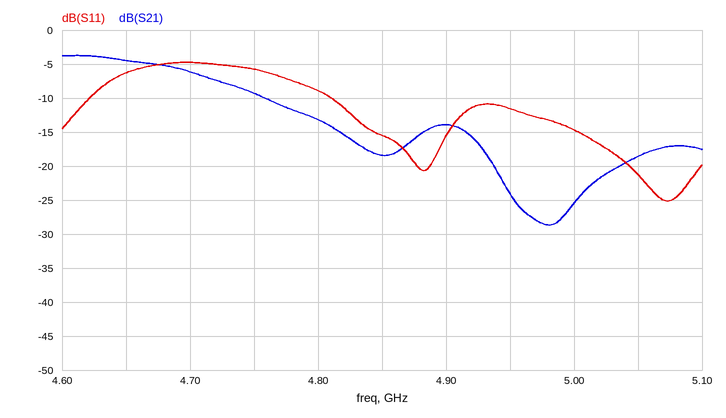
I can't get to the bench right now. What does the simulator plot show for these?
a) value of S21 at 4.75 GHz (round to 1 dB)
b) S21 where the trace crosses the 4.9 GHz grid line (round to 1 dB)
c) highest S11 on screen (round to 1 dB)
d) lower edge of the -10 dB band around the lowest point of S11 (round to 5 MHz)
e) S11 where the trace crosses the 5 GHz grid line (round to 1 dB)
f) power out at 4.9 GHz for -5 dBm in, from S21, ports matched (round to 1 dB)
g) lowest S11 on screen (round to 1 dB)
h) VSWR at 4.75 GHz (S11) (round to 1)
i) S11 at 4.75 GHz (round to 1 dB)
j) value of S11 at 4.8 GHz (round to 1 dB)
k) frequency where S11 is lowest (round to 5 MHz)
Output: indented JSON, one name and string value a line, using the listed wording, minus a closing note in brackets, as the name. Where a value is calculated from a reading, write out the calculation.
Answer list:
{
  "value of S21 at 4.75 GHz": "-9 dB",
  "S21 where the trace crosses the 4.9 GHz grid line": "-14 dB",
  "highest S11 on screen": "-5 dB",
  "lower edge of the -10 dB band around the lowest point of S11": "4.810 GHz",
  "S11 where the trace crosses the 5 GHz grid line": "-15 dB",
  "power out at 4.9 GHz for -5 dBm in, from S21, ports matched": "-5 dBm + (-14 dB) = -19 dBm",
  "lowest S11 on screen": "-25 dB",
  "VSWR at 4.75 GHz (S11)": "|Γ| = 10^(-6/20) = 0.5012; VSWR = (1 + 0.5012)/(1 − 0.5012) ≈ 3",
  "S11 at 4.75 GHz": "-6 dB",
  "value of S11 at 4.8 GHz": "-9 dB",
  "frequency where S11 is lowest": "5.075 GHz"
}
